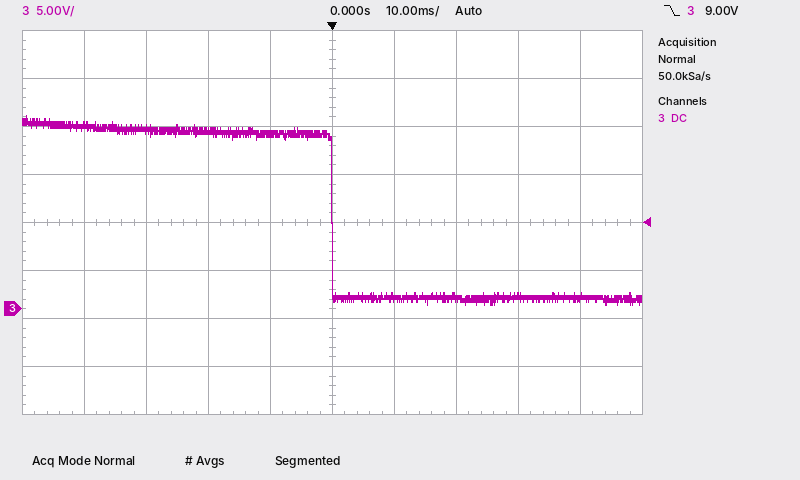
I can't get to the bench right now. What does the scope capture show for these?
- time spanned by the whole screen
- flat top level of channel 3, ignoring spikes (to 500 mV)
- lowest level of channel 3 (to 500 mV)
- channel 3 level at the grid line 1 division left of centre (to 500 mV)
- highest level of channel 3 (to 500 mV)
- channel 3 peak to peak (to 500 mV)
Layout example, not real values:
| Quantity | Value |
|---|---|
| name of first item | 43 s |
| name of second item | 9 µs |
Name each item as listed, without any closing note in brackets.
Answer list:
| Quantity | Value |
|---|---|
| time spanned by the whole screen | 100 ms |
| flat top level of channel 3, ignoring spikes | 18.5 V |
| lowest level of channel 3 | 500 mV |
| channel 3 level at the grid line 1 division left of centre | 18.5 V |
| highest level of channel 3 | 20.0 V |
| channel 3 peak to peak | 19.5 V |
